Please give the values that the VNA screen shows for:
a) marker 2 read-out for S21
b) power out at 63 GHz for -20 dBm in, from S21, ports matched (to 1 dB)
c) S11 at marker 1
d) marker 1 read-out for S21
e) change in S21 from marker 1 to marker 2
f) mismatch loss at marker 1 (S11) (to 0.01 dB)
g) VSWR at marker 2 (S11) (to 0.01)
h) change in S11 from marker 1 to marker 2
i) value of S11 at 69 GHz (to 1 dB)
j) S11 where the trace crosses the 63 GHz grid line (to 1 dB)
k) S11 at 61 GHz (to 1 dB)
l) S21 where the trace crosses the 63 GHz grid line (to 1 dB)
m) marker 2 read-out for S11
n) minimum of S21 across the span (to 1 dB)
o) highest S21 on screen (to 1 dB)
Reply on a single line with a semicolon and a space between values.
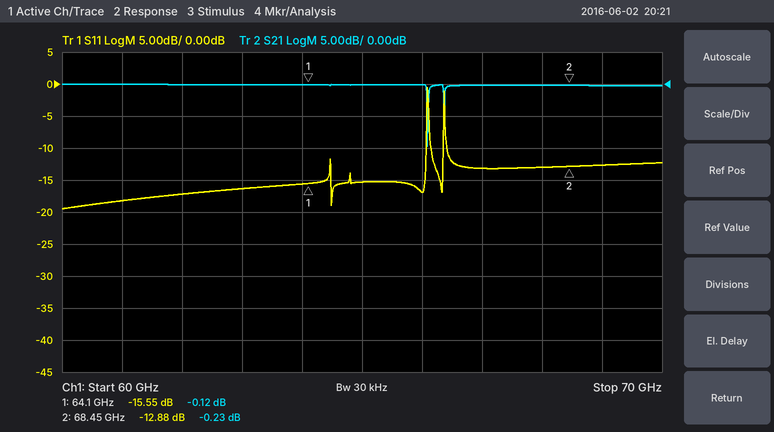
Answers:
-0.23 dB; -20 dBm; -15.55 dB; -0.12 dB; -0.11 dB; 0.12 dB; 1.59; 2.67 dB; -13 dB; -16 dB; -18 dB; 0 dB; -12.88 dB; -10 dB; 0 dB
